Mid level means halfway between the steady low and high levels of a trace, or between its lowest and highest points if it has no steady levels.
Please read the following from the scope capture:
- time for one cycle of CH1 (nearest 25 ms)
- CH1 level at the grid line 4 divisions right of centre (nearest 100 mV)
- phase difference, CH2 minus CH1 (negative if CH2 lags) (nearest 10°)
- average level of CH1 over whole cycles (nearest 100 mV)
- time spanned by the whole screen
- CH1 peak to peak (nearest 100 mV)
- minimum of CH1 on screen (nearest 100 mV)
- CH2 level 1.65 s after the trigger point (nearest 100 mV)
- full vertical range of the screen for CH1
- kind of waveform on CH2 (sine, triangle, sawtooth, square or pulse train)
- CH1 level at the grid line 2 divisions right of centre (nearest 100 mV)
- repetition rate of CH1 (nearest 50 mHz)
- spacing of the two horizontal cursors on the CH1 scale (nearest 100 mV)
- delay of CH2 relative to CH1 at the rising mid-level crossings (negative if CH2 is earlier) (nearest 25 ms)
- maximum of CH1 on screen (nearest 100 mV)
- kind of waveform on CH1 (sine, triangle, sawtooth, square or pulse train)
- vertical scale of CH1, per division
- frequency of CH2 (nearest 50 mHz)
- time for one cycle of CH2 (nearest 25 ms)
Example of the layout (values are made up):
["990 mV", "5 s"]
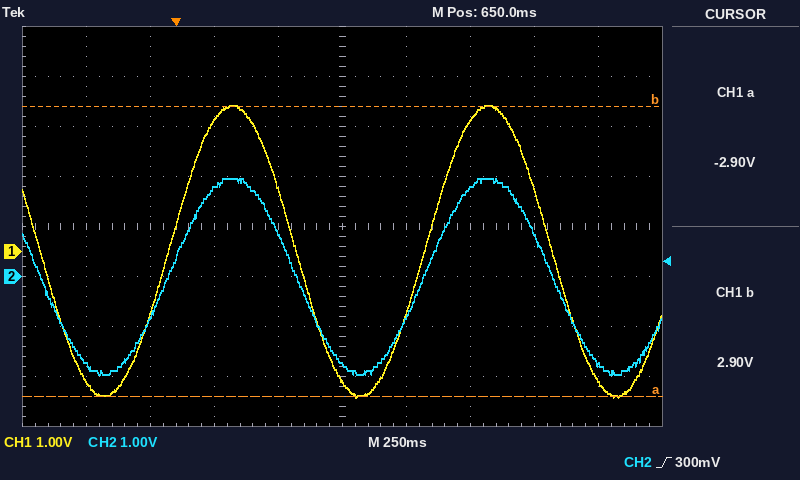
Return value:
["1.000 s", "-2.6 V", "0°", "0.0 V", "2.5 s", "5.8 V", "-2.9 V", "-1.7 V", "8 V", "sine", "2.6 V", "1.00 Hz", "5.8 V", "0 ms", "2.9 V", "sine", "1 V", "1.00 Hz", "1.000 s"]
